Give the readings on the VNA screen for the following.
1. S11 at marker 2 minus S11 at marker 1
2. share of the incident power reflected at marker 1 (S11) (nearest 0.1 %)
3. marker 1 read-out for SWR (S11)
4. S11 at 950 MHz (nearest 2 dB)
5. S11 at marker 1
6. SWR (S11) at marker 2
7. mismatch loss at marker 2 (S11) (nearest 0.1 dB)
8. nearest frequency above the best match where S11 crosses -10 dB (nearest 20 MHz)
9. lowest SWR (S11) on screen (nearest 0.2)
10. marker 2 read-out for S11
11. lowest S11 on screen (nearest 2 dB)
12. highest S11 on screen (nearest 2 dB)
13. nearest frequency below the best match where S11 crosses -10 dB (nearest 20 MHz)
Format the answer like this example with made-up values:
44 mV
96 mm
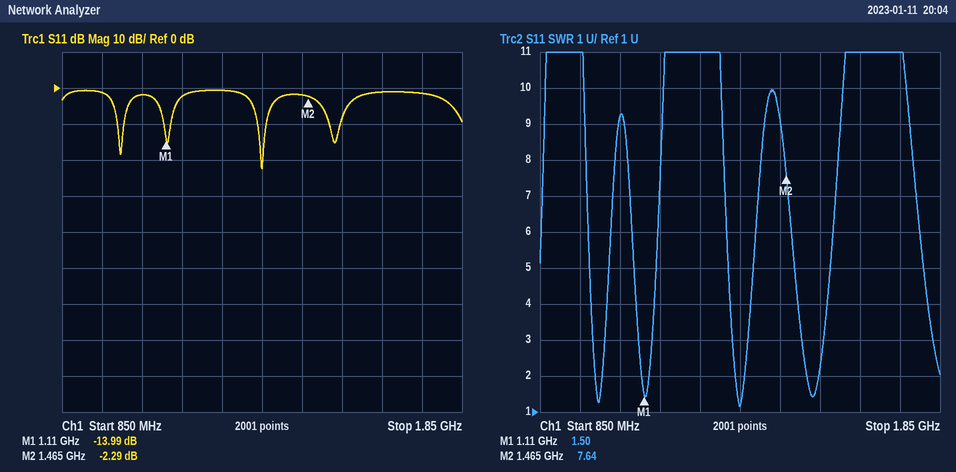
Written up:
11.70 dB
4.0 %
1.50
-2 dB
-13.99 dB
7.64
3.9 dB
1.36 GHz
1.2
-2.29 dB
-22 dB
0 dB
1.34 GHz
